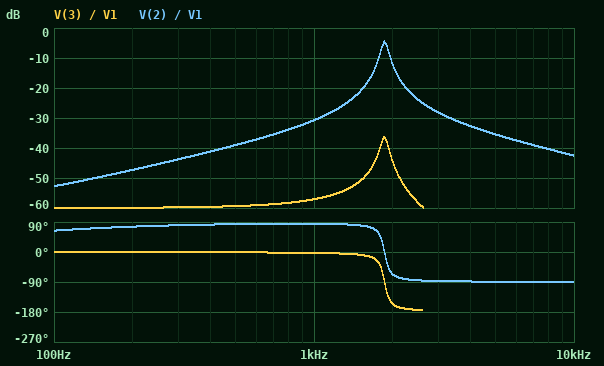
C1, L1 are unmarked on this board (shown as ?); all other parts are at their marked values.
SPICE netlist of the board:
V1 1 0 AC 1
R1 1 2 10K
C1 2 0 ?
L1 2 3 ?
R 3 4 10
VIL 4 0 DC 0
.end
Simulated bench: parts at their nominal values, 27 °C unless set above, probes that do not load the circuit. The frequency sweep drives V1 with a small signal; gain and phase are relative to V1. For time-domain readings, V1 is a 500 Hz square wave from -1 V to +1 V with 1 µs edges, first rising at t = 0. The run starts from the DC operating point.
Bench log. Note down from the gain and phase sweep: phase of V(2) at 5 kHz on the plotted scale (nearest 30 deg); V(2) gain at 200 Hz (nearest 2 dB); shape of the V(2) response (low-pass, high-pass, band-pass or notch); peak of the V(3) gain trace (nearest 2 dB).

-90 deg
-48 dB
band-pass
-36 dB
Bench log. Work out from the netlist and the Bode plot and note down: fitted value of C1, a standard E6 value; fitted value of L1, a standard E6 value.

220 nF
33 mH
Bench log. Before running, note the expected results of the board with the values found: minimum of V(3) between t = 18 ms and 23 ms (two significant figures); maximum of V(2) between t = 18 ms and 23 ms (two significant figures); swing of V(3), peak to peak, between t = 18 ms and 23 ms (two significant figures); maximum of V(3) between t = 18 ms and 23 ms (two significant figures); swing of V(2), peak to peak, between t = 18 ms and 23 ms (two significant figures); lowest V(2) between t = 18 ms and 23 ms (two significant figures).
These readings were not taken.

-2.2 mV
49 mV
4.4 mV
2.2 mV
98 mV
-49 mV
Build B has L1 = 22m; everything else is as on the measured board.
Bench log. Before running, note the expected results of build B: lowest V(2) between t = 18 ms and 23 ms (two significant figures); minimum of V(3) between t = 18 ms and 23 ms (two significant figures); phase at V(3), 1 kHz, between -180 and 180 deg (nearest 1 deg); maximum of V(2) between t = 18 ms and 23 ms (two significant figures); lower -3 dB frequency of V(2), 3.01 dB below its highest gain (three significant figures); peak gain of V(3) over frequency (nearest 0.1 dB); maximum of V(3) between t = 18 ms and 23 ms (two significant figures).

-57 mV
-2.7 mV
-2 deg
57 mV
2.22 kHz
-36.0 dB
2.7 mV
